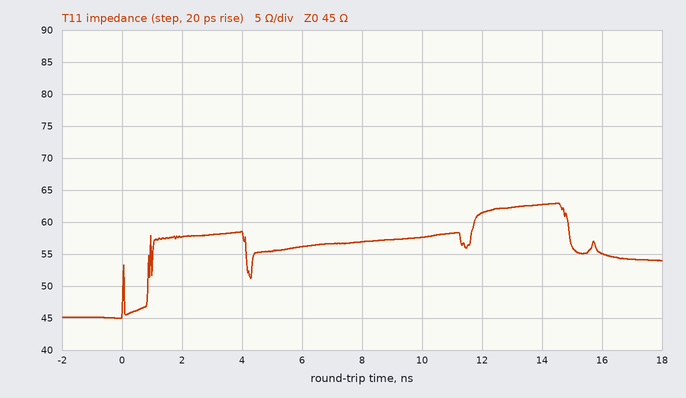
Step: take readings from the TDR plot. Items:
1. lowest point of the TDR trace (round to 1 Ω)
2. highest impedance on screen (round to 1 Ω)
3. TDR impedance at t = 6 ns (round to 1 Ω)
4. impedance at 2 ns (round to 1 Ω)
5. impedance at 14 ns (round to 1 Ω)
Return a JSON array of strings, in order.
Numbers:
["45 Ω", "63 Ω", "56 Ω", "58 Ω", "63 Ω"]
